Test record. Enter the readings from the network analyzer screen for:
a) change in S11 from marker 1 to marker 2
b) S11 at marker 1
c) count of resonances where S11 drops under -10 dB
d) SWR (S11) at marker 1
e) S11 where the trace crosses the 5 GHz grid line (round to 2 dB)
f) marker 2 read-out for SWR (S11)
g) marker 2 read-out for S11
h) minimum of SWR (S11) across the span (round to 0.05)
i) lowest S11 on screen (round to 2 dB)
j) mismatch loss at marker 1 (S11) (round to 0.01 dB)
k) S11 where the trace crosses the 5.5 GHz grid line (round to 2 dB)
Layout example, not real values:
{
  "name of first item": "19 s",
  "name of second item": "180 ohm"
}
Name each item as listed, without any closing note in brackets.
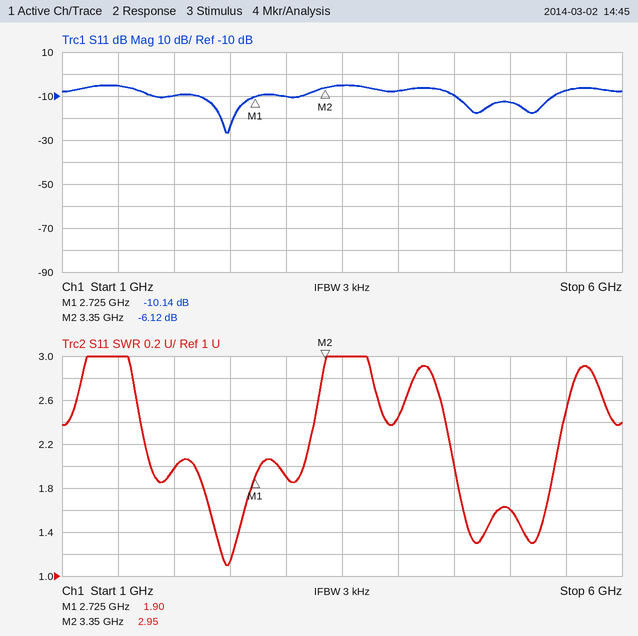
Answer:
{
  "change in S11 from marker 1 to marker 2": "4.02 dB",
  "S11 at marker 1": "-10.14 dB",
  "count of resonances where S11 drops under -10 dB": "3",
  "SWR (S11) at marker 1": "1.90",
  "S11 where the trace crosses the 5 GHz grid line": "-12 dB",
  "marker 2 read-out for SWR": "2.95",
  "marker 2 read-out for S11": "-6.12 dB",
  "minimum of SWR (S11) across the span": "1.10",
  "lowest S11 on screen": "-26 dB",
  "mismatch loss at marker 1 (S11)": "0.44 dB",
  "S11 where the trace crosses the 5.5 GHz grid line": "-8 dB"
}
